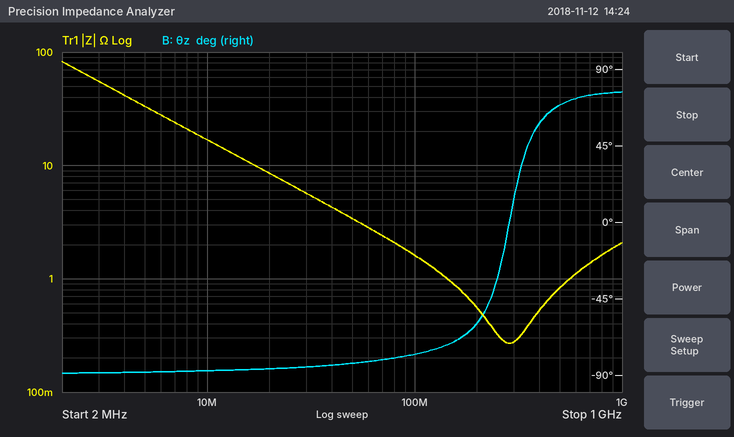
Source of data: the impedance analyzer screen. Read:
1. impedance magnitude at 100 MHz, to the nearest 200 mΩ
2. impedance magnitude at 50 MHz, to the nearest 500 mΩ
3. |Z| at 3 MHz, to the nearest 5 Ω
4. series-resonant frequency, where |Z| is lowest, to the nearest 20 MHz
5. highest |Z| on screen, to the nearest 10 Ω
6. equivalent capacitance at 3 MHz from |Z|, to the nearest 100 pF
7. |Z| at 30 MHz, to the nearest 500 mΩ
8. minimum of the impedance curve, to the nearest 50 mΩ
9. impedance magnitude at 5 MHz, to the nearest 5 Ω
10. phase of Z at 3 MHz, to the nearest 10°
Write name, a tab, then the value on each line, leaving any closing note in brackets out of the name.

impedance magnitude at 100 MHz, to the nearest 200 mΩ	1.6 Ω
impedance magnitude at 50 MHz, to the nearest 500 mΩ	3.5 Ω
|Z| at 3 MHz, to the nearest 5 Ω	55 Ω
series-resonant frequency, where |Z| is lowest, to the nearest 20 MHz	280 MHz
highest |Z| on screen, to the nearest 10 Ω	80 Ω
equivalent capacitance at 3 MHz from |Z|, to the nearest 100 pF	1.0 nF
|Z| at 30 MHz, to the nearest 500 mΩ	5.5 Ω
minimum of the impedance curve, to the nearest 50 mΩ	250 mΩ
impedance magnitude at 5 MHz, to the nearest 5 Ω	35 Ω
phase of Z at 3 MHz, to the nearest 10°	-90°
